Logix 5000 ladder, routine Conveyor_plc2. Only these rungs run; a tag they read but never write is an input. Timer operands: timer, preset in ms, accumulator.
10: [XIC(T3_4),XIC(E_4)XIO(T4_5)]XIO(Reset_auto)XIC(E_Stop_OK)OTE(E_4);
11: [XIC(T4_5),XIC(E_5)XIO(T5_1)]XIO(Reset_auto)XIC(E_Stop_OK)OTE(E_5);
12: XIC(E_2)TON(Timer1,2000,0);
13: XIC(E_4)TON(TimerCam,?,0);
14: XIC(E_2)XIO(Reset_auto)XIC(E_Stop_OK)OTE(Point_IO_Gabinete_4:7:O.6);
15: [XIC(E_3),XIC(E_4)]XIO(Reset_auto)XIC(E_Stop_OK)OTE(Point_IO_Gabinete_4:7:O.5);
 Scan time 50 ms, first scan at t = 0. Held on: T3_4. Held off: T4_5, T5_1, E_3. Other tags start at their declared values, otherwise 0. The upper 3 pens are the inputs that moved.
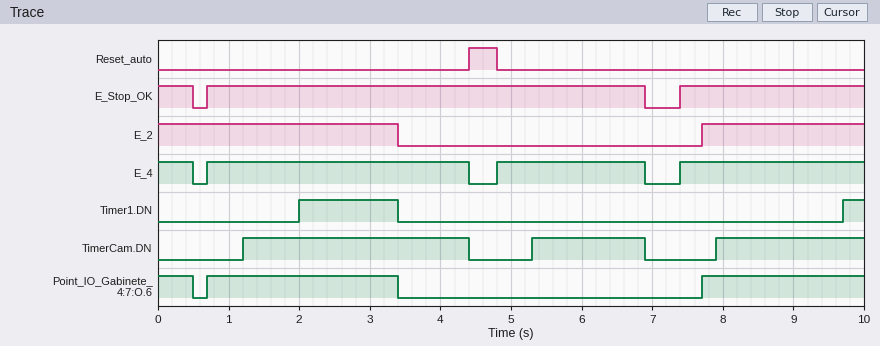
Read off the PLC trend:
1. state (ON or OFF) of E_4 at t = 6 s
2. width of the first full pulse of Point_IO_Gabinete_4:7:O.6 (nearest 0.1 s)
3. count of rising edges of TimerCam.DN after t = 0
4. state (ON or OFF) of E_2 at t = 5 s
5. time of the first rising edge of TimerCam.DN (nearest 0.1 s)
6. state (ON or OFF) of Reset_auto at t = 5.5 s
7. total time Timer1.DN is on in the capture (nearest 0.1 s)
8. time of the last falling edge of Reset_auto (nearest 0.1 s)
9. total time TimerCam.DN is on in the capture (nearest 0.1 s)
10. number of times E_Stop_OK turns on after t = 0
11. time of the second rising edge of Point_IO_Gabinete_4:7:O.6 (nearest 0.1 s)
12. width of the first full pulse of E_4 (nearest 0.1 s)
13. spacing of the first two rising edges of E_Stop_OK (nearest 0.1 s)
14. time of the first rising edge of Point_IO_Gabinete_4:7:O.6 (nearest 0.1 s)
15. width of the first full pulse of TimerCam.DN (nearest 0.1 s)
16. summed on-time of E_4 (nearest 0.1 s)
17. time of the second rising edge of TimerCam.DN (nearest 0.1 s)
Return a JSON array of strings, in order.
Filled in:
["ON", "2.7 s", "3", "OFF", "1.2 s", "OFF", "1.7 s", "4.8 s", "6.9 s", "2", "7.7 s", "3.7 s", "6.7 s", "0.7 s", "3.2 s", "8.9 s", "5.3 s"]
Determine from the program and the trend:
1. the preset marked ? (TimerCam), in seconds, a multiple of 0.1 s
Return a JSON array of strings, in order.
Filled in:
["0.5 s"]
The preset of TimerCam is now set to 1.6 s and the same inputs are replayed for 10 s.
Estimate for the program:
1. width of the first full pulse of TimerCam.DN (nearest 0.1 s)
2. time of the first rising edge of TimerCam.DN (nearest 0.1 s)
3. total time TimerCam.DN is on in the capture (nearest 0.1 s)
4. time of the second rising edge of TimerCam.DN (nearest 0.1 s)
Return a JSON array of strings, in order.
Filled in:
["2.1 s", "2.3 s", "3.6 s", "6.4 s"]
